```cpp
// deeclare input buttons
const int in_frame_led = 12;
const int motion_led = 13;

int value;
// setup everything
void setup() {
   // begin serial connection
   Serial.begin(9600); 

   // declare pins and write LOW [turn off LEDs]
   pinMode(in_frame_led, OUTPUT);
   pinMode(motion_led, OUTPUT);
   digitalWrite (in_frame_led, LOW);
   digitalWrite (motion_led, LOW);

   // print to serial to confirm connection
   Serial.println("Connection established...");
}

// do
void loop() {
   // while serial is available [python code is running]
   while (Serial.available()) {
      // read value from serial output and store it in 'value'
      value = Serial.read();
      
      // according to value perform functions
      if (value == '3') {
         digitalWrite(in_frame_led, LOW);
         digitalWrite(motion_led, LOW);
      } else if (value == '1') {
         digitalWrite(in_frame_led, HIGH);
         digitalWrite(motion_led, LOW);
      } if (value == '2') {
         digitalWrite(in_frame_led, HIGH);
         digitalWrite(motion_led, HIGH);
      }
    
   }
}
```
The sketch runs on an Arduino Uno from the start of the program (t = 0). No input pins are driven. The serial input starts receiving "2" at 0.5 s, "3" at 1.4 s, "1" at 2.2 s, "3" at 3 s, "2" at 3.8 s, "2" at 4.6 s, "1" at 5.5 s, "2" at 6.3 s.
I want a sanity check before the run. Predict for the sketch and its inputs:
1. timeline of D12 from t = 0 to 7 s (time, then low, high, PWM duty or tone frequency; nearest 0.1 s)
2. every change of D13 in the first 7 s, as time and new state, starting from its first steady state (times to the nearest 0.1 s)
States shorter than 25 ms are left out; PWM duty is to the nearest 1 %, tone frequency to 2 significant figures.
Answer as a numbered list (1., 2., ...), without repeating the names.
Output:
1. 0 s low; 0.5 s high; 1.4 s low; 2.2 s high; 3 s low; 3.8 s high
2. 0 s low; 0.5 s high; 1.4 s low; 3.8 s high; 5.5 s low; 6.3 s high
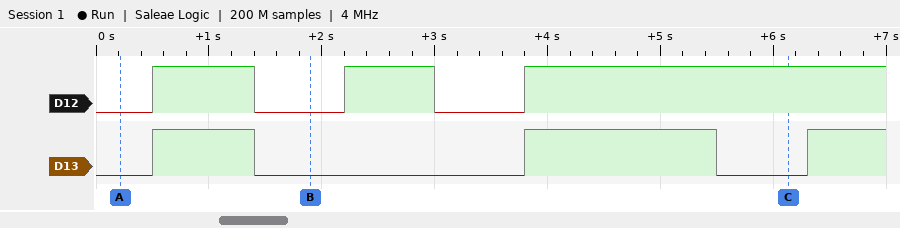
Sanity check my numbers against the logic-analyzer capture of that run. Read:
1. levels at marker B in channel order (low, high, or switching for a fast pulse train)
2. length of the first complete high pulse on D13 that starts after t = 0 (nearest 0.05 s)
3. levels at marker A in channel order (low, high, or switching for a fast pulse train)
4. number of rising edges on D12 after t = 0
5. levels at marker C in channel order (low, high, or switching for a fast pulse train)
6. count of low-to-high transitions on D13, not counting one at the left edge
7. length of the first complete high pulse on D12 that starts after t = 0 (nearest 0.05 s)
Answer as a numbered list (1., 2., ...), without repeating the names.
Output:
1. D12 low, D13 low
2. 0.90 s
3. D12 low, D13 low
4. 3
5. D12 high, D13 low
6. 3
7. 0.90 s
